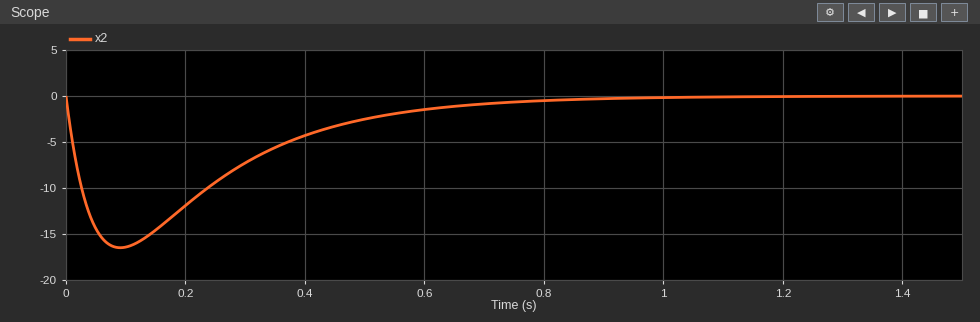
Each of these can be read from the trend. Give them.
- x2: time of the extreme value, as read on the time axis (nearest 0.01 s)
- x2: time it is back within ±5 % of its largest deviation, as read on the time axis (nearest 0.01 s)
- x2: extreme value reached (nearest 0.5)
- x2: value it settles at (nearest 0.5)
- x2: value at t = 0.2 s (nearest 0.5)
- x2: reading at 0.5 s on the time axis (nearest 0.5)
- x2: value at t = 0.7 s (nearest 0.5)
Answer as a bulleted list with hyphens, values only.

- 0.09 s
- 0.71 s
- -16.5
- 0.0
- -12.0
- -2.5
- -1.0
